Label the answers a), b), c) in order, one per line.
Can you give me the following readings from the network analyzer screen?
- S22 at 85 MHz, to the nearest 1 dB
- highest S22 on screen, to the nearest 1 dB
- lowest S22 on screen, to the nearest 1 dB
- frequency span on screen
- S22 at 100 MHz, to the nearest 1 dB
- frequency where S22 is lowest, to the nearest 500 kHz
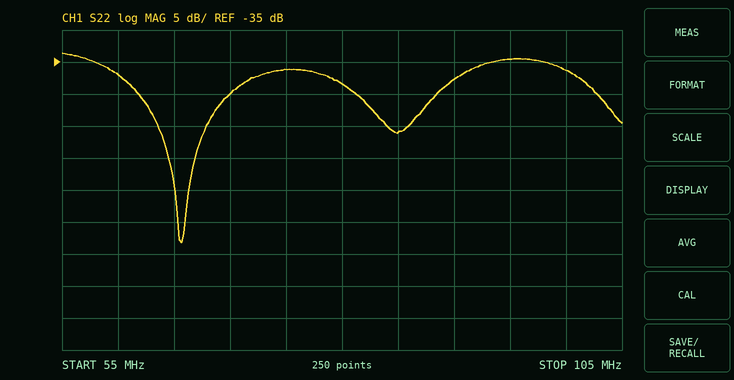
a) -46 dB
b) -34 dB
c) -63 dB
d) 50 MHz
e) -36 dB
f) 65.5 MHz
